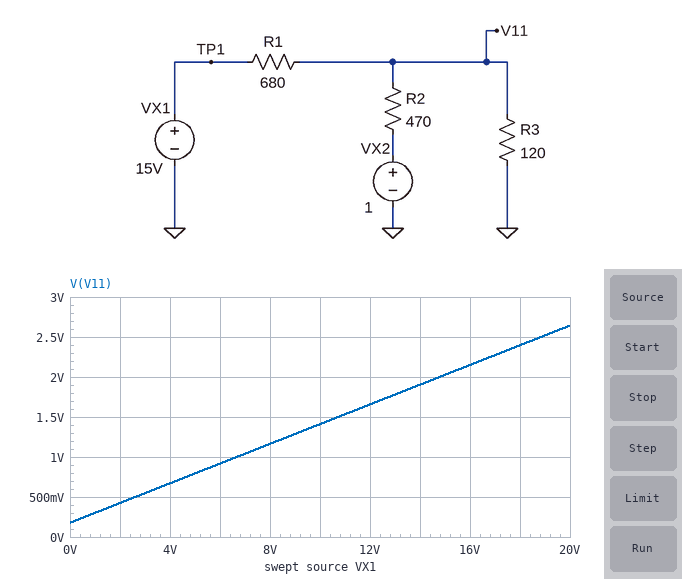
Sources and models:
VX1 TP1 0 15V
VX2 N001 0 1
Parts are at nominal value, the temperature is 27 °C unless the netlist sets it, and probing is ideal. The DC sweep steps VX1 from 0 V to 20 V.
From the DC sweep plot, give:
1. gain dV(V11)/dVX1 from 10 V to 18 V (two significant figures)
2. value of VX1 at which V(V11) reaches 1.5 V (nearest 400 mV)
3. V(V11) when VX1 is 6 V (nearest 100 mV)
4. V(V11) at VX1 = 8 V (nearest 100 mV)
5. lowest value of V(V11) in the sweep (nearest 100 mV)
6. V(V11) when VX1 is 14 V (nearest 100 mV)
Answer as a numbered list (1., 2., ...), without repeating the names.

1. 0.12 V/V
2. 10.8 V
3. 900 mV
4. 1.2 V
5. 200 mV
6. 1.9 V
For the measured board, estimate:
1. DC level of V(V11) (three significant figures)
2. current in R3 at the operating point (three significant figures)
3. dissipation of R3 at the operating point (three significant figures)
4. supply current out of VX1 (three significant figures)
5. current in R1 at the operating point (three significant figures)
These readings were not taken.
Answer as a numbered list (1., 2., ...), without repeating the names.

1. 2.03 V
2. 16.9 mA
3. 34.2 mW
4. 19.1 mA
5. 19.1 mA
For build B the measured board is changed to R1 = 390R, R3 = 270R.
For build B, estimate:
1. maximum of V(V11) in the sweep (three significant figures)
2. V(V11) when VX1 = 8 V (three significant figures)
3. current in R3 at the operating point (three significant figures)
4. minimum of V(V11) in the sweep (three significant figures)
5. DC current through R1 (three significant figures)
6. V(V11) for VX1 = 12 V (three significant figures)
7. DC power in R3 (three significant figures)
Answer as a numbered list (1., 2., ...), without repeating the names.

1. 6.36 V
2. 2.70 V
3. 17.9 mA
4. 253 mV
5. 26.1 mA
6. 3.92 V
7. 86.6 mW
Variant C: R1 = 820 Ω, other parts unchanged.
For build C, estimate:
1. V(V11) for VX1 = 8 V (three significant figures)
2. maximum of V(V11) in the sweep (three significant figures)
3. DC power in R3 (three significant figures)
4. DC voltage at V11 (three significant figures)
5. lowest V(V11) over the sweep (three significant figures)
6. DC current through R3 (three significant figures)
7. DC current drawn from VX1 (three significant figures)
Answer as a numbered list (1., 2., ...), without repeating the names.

1. 1.02 V
2. 2.27 V
3. 25.5 mW
4. 1.75 V
5. 182 mV
6. 14.6 mA
7. 16.2 mA
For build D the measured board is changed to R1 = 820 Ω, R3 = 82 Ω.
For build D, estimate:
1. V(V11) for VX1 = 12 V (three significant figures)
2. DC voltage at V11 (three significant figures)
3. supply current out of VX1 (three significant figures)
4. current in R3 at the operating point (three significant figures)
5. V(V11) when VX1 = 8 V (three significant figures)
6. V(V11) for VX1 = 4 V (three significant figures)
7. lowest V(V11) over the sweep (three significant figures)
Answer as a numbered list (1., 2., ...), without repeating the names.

1. 1.08 V
2. 1.31 V
3. 16.7 mA
4. 16.0 mA
5. 765 mV
6. 451 mV
7. 137 mV
